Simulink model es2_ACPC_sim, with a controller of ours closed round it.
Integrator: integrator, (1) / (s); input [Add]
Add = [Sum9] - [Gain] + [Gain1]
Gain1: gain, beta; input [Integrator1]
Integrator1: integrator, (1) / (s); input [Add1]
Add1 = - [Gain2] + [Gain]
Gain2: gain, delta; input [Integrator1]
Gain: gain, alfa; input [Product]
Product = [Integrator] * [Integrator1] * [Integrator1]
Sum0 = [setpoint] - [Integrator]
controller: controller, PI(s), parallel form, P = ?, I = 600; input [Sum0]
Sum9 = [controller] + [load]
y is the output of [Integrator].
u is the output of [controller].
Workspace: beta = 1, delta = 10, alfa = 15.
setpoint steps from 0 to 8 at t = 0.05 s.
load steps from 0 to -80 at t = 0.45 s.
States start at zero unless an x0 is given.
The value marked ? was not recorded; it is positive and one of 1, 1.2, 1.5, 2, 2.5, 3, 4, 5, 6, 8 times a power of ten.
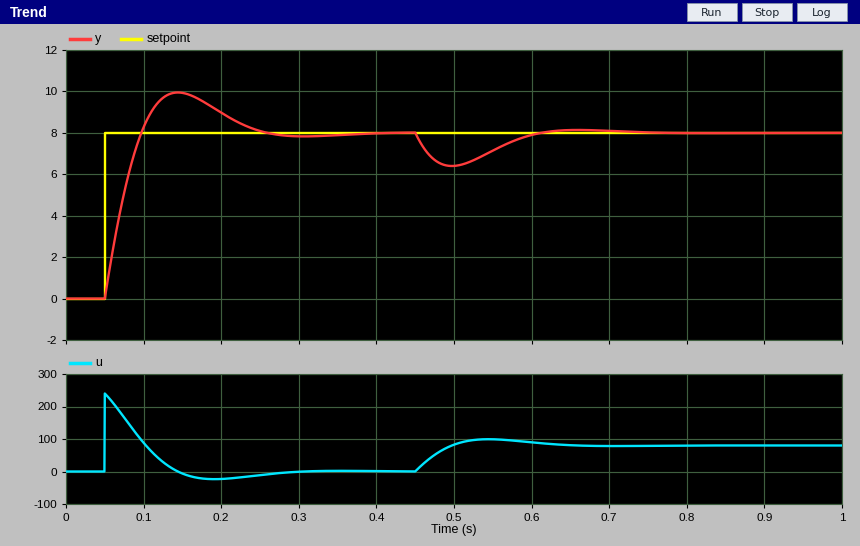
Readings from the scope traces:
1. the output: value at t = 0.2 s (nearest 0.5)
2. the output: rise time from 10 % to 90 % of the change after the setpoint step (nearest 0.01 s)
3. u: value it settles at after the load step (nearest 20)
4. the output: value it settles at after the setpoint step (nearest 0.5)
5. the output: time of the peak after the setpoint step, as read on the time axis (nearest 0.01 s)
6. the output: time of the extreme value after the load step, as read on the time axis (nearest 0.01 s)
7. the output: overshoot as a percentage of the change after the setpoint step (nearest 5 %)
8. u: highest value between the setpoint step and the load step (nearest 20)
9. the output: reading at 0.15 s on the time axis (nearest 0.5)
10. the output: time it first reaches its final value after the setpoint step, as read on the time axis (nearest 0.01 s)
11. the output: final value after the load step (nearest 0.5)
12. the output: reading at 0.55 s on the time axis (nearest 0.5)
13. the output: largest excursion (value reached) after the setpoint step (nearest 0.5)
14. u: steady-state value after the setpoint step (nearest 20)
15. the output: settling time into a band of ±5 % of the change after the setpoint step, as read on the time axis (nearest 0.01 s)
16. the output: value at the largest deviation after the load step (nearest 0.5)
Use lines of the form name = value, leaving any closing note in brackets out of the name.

the output: value at t = 0.2 s = 9.0
the output: rise time from 10 % to 90 % of the change after the setpoint step = 0.04 s
u: value it settles at after the load step = 80
the output: value it settles at after the setpoint step = 8.0
the output: time of the peak after the setpoint step, as read on the time axis = 0.14 s
the output: time of the extreme value after the load step, as read on the time axis = 0.50 s
the output: overshoot as a percentage of the change after the setpoint step = 25 %
u: highest value between the setpoint step and the load step = 240
the output: reading at 0.15 s on the time axis = 10.0
the output: time it first reaches its final value after the setpoint step, as read on the time axis = 0.10 s
the output: final value after the load step = 8.0
the output: reading at 0.55 s on the time axis = 7.0
the output: largest excursion (value reached) after the setpoint step = 10.0
u: steady-state value after the setpoint step = 0
the output: settling time into a band of ±5 % of the change after the setpoint step, as read on the time axis = 0.23 s
the output: value at the largest deviation after the load step = 6.5
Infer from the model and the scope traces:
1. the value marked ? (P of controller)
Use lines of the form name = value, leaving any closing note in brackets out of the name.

the value marked ? = 30
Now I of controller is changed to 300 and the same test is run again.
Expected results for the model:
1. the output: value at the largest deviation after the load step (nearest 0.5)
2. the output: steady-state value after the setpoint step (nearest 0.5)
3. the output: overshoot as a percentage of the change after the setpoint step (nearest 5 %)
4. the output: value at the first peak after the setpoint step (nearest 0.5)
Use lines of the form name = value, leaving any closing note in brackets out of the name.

the output: value at the largest deviation after the load step = 6.0
the output: steady-state value after the setpoint step = 8.0
the output: overshoot as a percentage of the change after the setpoint step = 15 %
the output: value at the first peak after the setpoint step = 9.5
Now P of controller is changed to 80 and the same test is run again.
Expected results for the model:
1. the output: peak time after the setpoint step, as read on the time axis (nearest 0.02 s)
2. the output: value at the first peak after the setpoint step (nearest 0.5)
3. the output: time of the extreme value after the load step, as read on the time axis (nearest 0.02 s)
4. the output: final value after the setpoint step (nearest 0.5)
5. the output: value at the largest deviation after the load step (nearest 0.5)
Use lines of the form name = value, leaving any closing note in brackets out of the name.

the output: peak time after the setpoint step, as read on the time axis = 0.12 s
the output: value at the first peak after the setpoint step = 8.5
the output: time of the extreme value after the load step, as read on the time axis = 0.48 s
the output: final value after the setpoint step = 8.0
the output: value at the largest deviation after the load step = 7.0
